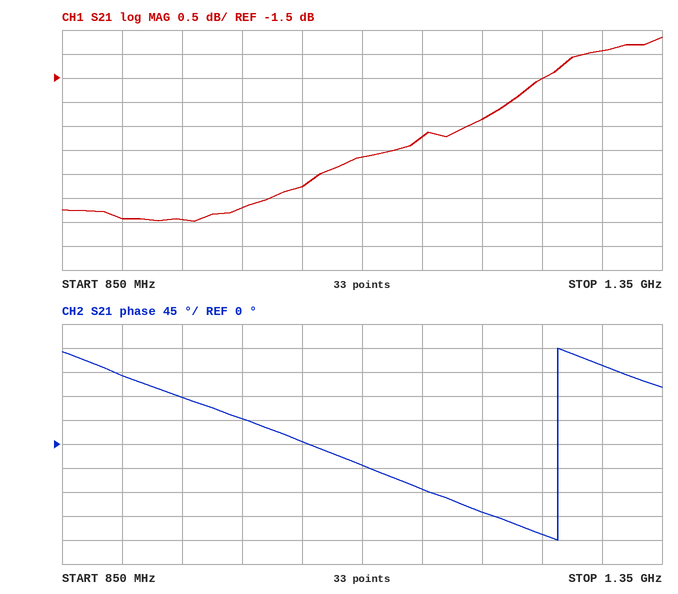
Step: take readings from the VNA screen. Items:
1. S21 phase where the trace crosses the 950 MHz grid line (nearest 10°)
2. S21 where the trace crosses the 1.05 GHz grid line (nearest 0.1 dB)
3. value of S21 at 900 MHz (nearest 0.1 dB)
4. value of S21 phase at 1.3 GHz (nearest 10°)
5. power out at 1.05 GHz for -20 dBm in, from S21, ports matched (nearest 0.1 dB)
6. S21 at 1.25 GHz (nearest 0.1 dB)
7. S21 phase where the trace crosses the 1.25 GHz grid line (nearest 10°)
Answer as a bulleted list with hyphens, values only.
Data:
- 90°
- -3.8 dB
- -4.4 dB
- 150°
- -23.8 dBm
- -1.5 dB
- -170°
